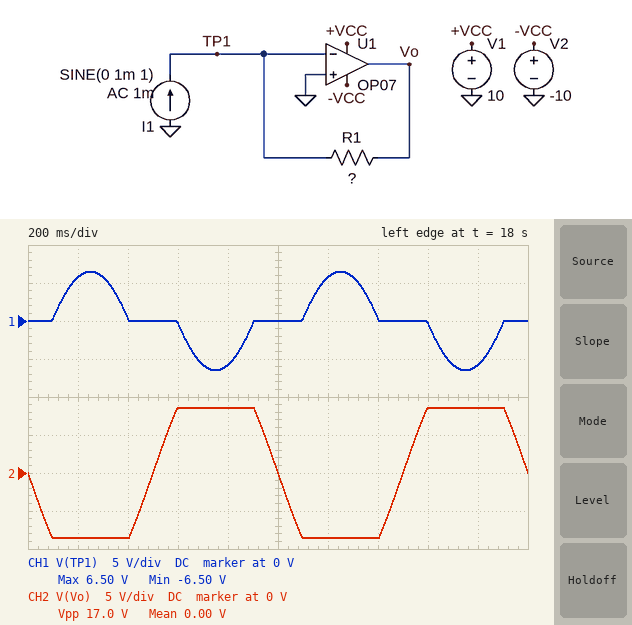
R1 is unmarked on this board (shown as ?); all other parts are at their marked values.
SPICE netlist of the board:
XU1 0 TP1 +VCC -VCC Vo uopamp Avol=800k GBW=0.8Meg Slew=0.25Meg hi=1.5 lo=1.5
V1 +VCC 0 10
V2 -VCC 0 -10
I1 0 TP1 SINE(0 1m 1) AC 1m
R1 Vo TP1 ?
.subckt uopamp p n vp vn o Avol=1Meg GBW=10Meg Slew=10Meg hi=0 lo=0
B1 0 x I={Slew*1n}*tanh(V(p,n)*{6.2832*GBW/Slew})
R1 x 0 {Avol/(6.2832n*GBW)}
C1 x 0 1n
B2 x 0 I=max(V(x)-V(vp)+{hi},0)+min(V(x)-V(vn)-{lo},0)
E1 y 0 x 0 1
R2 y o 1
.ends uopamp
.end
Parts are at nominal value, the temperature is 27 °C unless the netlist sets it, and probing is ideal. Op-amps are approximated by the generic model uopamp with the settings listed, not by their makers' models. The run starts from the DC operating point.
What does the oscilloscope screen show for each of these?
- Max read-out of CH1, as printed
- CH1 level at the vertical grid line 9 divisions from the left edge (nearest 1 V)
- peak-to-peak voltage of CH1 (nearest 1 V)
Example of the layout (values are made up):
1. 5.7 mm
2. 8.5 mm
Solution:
1. 6.50 V
2. -6 V
3. 13 V
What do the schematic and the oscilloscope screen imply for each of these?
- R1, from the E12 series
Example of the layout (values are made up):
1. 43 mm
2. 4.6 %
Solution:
1. 15 kΩ
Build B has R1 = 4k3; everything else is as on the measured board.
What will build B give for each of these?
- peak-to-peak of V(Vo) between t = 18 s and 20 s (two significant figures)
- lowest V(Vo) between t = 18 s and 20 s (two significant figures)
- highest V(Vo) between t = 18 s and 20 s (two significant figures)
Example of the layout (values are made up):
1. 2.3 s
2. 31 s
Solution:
1. 8.6 V
2. -4.3 V
3. 4.3 V
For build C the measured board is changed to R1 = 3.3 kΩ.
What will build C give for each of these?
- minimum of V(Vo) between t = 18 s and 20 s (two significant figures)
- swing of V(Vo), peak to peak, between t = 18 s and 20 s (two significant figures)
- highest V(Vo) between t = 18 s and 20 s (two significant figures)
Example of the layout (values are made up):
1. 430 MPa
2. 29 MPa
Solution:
1. -3.3 V
2. 6.6 V
3. 3.3 V
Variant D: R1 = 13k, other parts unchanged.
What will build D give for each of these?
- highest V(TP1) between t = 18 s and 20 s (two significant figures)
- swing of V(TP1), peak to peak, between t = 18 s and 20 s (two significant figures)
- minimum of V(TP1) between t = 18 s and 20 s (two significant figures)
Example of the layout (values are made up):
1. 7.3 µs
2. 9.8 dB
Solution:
1. 4.5 V
2. 9.0 V
3. -4.5 V
